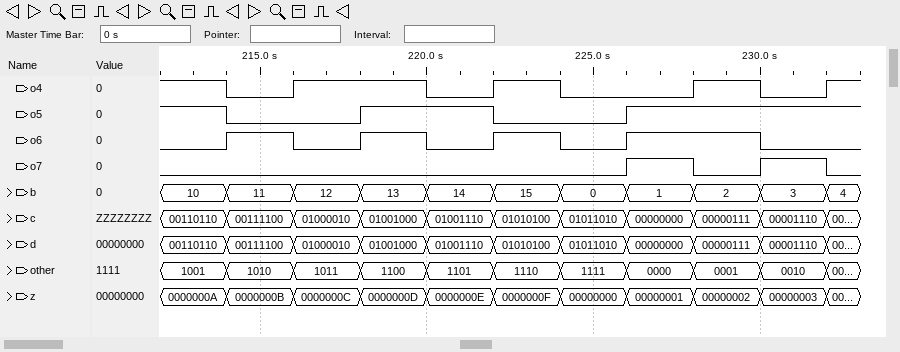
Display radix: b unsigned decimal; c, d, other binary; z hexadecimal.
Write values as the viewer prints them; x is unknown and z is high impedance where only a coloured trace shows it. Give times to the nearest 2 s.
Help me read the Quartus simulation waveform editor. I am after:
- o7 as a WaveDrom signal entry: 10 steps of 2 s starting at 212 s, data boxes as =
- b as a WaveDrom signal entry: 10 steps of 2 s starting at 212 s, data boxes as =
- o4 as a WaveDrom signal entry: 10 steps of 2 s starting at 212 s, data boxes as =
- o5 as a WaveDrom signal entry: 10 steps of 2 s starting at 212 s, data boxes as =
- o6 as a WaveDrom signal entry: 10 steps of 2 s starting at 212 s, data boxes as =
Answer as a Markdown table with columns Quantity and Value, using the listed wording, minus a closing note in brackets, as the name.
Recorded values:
| Quantity | Value |
|---|---|
| o7 as a WaveDrom signal entry: 10 steps of 2 s starting at 212 s, data boxes as = | {name: 'o7', wave: '0......101'} |
| b as a WaveDrom signal entry: 10 steps of 2 s starting at 212 s, data boxes as = | {name: 'b', wave: '==========', data: '10 11 12 13 14 15 0 1 2 3'} |
| o4 as a WaveDrom signal entry: 10 steps of 2 s starting at 212 s, data boxes as = | {name: 'o4', wave: '101.010.10'} |
| o5 as a WaveDrom signal entry: 10 steps of 2 s starting at 212 s, data boxes as = | {name: 'o5', wave: '10.1.0.1..'} |
| o6 as a WaveDrom signal entry: 10 steps of 2 s starting at 212 s, data boxes as = | {name: 'o6', wave: '01010101.0'} |
